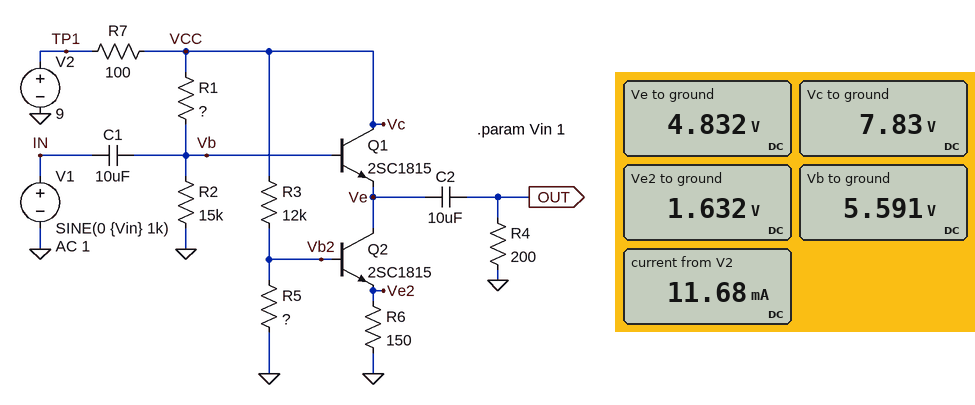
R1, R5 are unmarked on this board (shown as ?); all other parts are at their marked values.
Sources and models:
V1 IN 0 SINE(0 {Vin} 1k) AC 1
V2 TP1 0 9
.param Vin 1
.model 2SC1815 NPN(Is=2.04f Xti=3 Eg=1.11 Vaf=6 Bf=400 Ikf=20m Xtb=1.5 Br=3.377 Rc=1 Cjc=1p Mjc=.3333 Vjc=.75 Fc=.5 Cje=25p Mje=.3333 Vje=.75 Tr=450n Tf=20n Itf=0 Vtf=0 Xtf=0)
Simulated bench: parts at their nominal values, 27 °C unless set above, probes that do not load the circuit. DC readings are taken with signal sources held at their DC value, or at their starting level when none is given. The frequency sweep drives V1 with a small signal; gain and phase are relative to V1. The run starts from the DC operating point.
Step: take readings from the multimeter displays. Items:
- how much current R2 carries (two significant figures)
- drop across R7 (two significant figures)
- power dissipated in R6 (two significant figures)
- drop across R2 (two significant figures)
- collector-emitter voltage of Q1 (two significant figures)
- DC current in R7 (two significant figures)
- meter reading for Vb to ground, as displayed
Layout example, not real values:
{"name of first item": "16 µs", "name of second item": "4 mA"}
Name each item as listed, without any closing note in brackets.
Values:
{"how much current R2 carries": "370 µA", "drop across R7": "1.2 V", "power dissipated in R6": "18 mW", "drop across R2": "5.6 V", "collector-emitter voltage of Q1": "3.0 V", "DC current in R7": "12 mA", "meter reading for Vb to ground, as displayed": "5.591 V"}
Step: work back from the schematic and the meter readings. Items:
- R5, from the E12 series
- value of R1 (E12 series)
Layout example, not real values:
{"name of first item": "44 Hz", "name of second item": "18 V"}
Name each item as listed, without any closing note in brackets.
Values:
{"R5, from the E12 series": "5.6 kΩ", "value of R1": "5.6 kΩ"}
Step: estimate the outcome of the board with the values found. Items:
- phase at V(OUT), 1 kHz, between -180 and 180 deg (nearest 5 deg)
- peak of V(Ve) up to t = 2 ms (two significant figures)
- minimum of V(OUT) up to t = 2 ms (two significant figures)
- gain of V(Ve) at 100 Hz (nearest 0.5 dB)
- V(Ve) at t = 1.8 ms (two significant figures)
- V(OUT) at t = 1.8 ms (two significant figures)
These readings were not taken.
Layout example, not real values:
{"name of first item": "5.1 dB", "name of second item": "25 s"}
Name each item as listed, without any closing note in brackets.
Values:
{"phase at V(OUT), 1 kHz, between -180 and 180 deg": "5 deg", "peak of V(Ve) up to t = 2 ms": "5.8 V", "minimum of V(OUT) up to t = 2 ms": "-1.0 V", "gain of V(Ve) at 100 Hz": "0 dB", "V(Ve) at t = 1.8 ms": "3.9 V", "V(OUT) at t = 1.8 ms": "-930 mV"}
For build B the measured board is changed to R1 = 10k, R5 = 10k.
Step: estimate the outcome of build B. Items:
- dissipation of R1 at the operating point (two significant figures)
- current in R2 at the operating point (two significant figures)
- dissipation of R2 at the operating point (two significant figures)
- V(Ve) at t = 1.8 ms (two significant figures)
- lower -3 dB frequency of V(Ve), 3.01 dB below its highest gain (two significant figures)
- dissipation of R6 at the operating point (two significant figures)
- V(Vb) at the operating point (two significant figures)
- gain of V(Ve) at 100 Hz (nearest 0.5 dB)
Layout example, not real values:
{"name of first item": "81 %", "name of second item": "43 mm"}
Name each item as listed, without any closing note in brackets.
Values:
{"dissipation of R1 at the operating point": "1.0 mW", "current in R2 at the operating point": "280 µA", "dissipation of R2 at the operating point": "1.2 mW", "V(Ve) at t = 1.8 ms": "2.5 V", "lower -3 dB frequency of V(Ve), 3.01 dB below its highest gain": "2.8 Hz", "dissipation of R6 at the operating point": "34 mW", "V(Vb) at the operating point": "4.2 V", "gain of V(Ve) at 100 Hz": "0 dB"}
